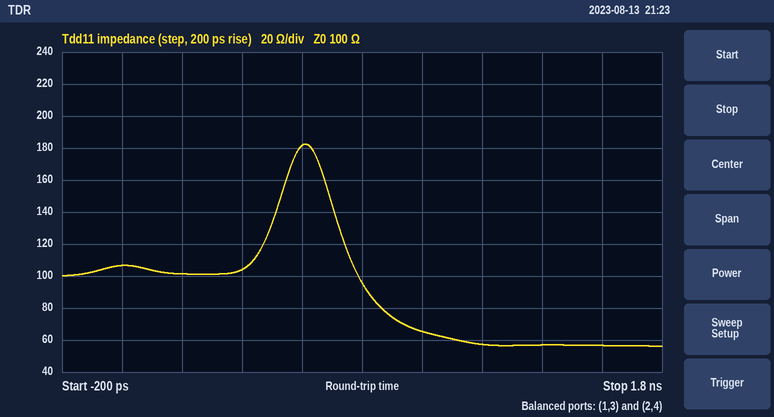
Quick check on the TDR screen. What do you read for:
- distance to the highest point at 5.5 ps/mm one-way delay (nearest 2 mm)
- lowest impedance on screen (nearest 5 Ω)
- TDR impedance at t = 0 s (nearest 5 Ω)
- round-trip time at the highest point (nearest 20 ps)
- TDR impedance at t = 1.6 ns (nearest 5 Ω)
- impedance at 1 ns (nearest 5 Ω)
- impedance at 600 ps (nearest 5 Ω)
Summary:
56 mm
55 Ω
105 Ω
620 ps
55 Ω
65 Ω
180 Ω
